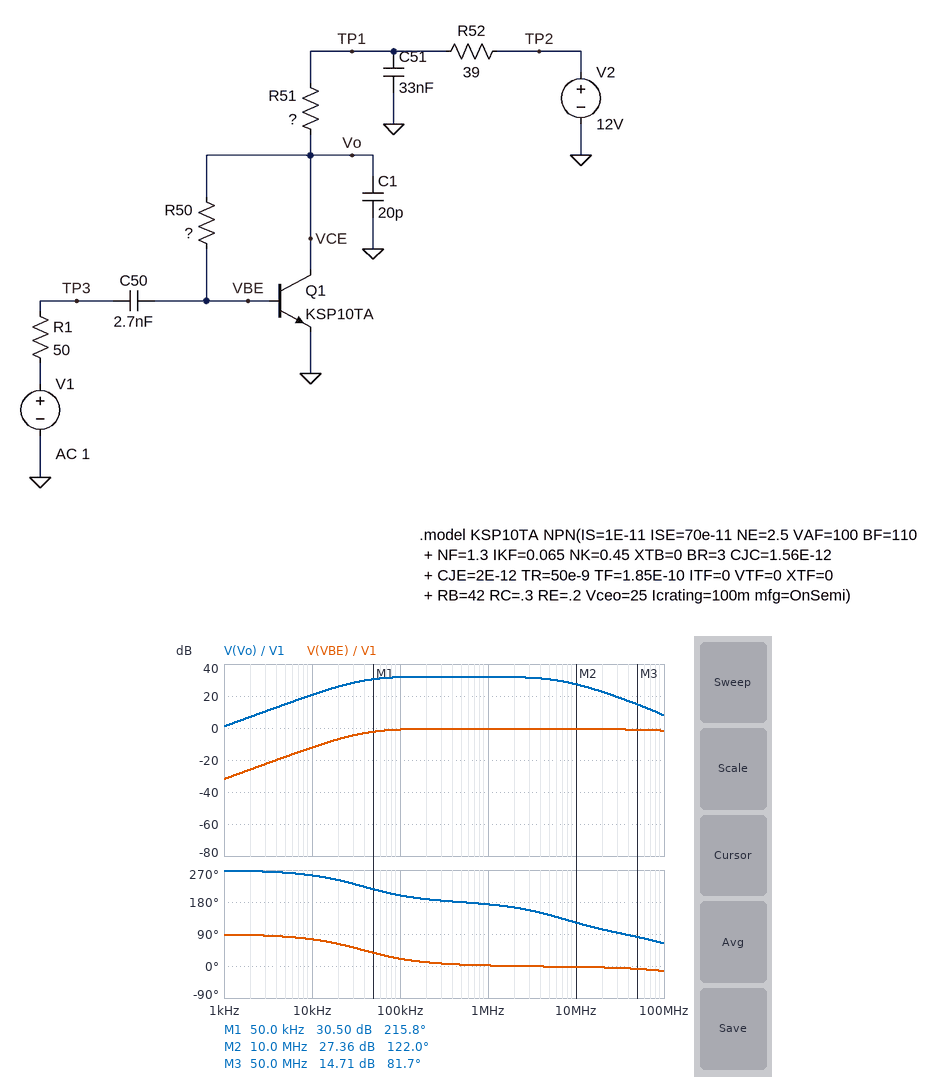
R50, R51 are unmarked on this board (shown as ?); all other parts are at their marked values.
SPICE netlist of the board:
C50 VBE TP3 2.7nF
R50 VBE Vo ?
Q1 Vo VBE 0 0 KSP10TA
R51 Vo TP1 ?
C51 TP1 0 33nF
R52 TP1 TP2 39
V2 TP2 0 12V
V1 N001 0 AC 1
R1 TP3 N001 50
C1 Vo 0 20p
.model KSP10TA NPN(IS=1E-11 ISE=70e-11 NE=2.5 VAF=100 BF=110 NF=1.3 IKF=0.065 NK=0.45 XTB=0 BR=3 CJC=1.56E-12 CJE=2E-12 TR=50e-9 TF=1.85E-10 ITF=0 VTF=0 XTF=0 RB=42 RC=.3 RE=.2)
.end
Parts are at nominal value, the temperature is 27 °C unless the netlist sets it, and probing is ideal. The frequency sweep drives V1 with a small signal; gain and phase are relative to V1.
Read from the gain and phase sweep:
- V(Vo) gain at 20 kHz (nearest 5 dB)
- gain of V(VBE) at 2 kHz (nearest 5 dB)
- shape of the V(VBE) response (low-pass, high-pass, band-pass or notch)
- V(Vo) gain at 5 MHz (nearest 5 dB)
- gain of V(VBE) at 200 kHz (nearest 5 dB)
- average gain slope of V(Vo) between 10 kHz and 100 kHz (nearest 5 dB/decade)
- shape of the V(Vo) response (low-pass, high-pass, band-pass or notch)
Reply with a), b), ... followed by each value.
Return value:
a) 25 dB
b) -25 dB
c) high-pass
d) 30 dB
e) 0 dB
f) 10 dB/decade
g) band-pass
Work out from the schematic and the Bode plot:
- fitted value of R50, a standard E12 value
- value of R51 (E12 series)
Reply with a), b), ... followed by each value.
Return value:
a) 390 kΩ
b) 1 kΩ
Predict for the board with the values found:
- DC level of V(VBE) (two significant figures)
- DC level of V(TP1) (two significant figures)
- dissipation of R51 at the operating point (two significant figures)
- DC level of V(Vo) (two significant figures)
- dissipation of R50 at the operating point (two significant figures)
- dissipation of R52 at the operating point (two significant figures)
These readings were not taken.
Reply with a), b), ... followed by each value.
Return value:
a) 630 mV
b) 12 V
c) 2.4 mW
d) 10 V
e) 240 µW
f) 94 µW
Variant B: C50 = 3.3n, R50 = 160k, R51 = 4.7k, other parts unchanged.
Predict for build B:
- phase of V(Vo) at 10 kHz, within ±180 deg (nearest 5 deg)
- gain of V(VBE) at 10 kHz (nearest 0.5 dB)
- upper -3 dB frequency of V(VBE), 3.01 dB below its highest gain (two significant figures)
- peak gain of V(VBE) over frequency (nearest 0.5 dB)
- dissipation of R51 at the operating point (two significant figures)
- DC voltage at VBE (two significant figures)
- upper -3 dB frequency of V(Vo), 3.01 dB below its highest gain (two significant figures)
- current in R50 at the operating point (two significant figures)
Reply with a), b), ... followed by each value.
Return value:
a) -100 deg
b) -18.5 dB
c) 250 MHz
d) -1.0 dB
e) 11 mW
f) 630 mV
g) 1.8 MHz
h) 26 µA
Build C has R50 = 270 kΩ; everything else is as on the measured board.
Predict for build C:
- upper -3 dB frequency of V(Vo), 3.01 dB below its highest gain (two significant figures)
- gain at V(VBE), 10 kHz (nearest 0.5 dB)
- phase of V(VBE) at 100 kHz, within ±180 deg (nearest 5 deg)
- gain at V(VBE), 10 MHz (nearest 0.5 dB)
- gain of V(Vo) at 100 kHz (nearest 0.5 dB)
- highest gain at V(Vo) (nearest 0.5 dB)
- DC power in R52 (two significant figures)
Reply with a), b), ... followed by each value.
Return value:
a) 6.9 MHz
b) -15.5 dB
c) 30 deg
d) -1.0 dB
e) 34.0 dB
f) 35.0 dB
g) 190 µW
